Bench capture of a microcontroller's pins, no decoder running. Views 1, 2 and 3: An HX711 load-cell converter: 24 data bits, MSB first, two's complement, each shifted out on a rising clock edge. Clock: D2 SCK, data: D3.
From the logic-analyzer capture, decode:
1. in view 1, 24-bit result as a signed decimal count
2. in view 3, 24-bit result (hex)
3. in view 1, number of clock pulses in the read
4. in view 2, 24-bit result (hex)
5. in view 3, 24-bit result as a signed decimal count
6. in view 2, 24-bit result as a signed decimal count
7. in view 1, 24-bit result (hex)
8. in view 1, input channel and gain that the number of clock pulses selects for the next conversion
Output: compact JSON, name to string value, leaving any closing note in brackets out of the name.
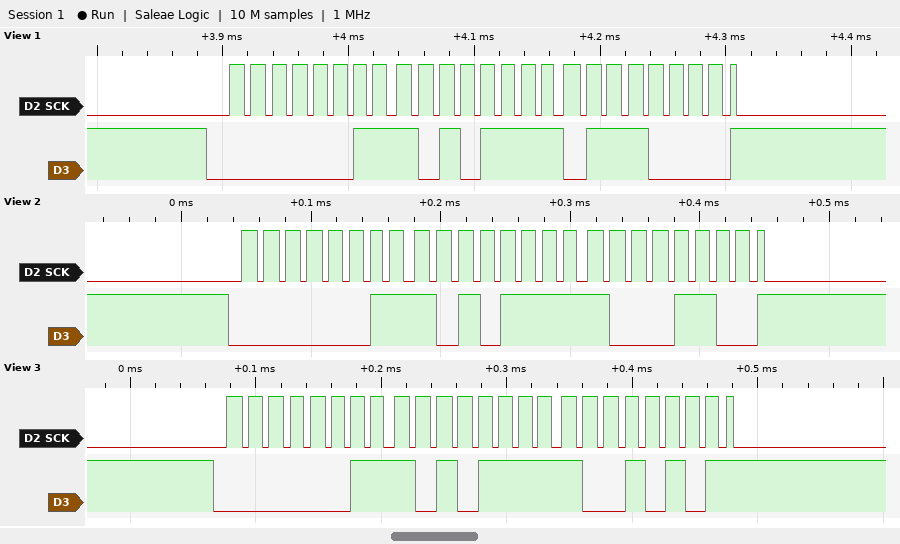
{"in view 1, 24-bit result as a signed decimal count": "241520", "in view 3, 24-bit result": "0x03AF95", "in view 1, number of clock pulses in the read": "25", "in view 2, 24-bit result": "0x03AF8C", "in view 3, 24-bit result as a signed decimal count": "241557", "in view 2, 24-bit result as a signed decimal count": "241548", "in view 1, 24-bit result": "0x03AF70", "in view 1, input channel and gain that the number of clock pulses selects for the next conversion": "channel A, gain 128"}
